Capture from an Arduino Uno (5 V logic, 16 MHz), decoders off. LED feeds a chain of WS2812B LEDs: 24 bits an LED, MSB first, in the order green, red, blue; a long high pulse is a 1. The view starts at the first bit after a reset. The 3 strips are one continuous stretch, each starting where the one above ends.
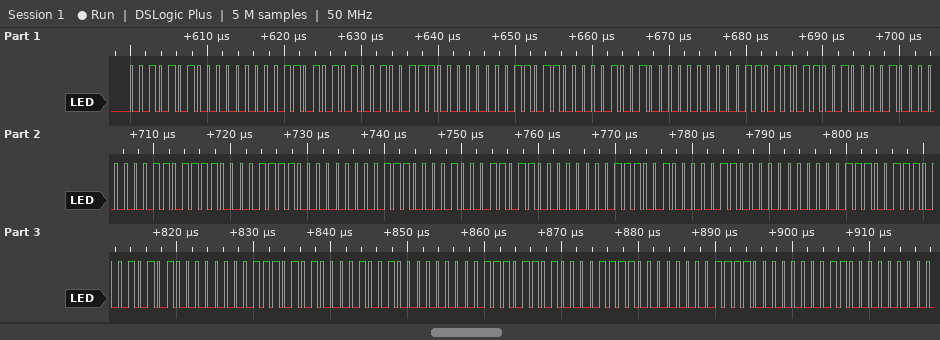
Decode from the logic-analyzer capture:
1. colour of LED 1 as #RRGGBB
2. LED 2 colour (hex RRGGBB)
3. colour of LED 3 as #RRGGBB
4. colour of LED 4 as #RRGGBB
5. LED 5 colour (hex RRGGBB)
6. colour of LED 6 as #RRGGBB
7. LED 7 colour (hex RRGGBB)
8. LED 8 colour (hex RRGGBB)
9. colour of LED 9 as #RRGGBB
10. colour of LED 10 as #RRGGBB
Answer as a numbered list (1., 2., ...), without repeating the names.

1. #002AD5
2. #0027D8
3. #0024DB
4. #0021DE
5. #001EE1
6. #001BE4
7. #0018E7
8. #0015EA
9. #0012ED
10. #000FF0
